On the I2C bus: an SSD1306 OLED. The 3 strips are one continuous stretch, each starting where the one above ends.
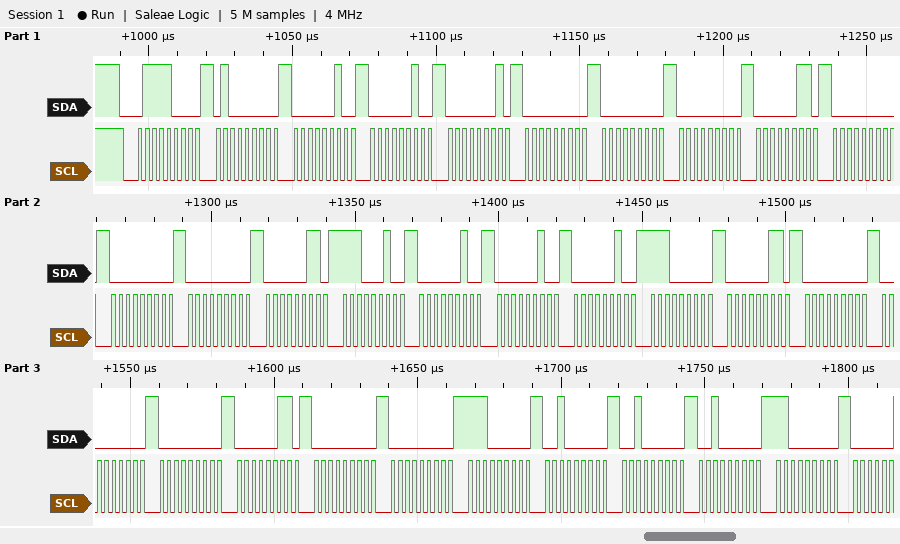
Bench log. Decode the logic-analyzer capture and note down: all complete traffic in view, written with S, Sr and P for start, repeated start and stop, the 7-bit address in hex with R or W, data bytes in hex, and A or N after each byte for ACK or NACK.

S 3CW A 40 A 02 A 02 A 01 A 00 A 00 A 00 A 03 A 00 A 00 A 00 A 03 A E2 A 02 A 02 A 02 A E0 A 03 A 00 A 00 A 00 A 03 A 00 A 00 A E0 A 20 A 20 A 20 A C0 A
